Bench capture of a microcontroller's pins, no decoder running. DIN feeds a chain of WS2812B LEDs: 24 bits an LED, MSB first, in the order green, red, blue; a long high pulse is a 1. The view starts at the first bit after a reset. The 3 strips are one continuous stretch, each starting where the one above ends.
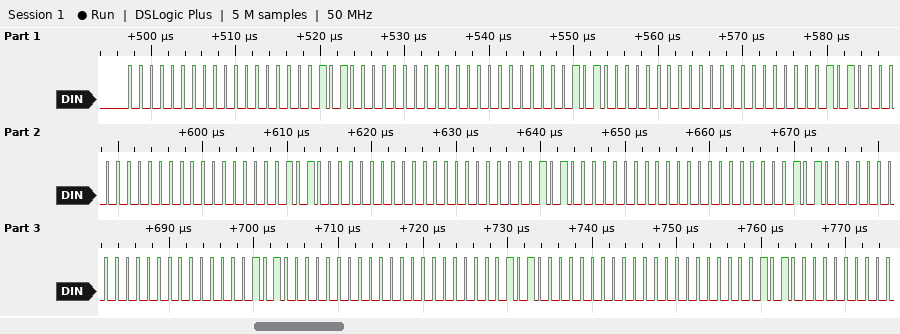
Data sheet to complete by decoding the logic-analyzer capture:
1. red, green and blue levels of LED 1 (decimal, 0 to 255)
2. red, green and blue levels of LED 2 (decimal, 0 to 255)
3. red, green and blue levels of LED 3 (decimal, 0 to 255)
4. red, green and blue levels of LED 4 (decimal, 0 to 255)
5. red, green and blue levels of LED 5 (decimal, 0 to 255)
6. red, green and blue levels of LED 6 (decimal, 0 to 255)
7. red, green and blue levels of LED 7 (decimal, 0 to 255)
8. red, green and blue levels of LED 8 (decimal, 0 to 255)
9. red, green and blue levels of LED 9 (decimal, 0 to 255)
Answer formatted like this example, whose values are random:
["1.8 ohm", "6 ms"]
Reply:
["0, 0, 40", "0, 0, 40", "0, 0, 40", "0, 0, 40", "0, 0, 40", "0, 0, 40", "0, 0, 40", "0, 0, 40", "0, 0, 40"]
